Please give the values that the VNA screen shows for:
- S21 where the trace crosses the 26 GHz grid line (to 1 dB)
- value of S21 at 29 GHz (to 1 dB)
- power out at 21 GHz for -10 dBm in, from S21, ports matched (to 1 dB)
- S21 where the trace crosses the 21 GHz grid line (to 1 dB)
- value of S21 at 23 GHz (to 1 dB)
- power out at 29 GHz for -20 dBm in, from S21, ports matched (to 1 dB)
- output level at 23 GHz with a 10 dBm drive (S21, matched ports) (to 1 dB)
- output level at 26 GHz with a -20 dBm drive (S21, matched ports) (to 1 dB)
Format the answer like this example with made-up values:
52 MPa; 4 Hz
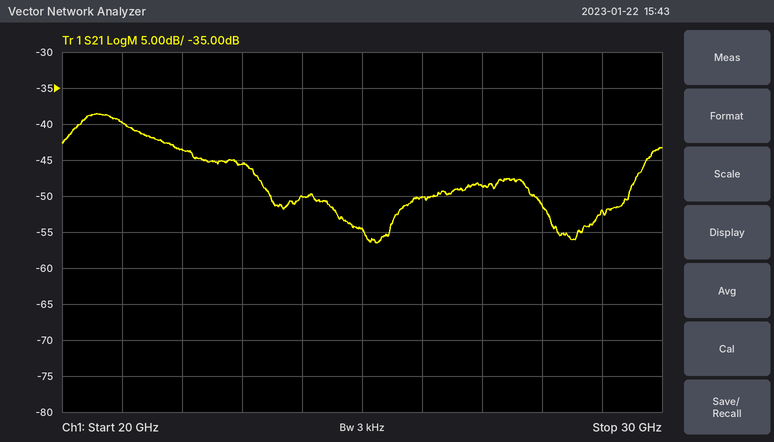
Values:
-50 dB; -52 dB; -50 dBm; -40 dB; -46 dB; -72 dBm; -36 dBm; -70 dBm
